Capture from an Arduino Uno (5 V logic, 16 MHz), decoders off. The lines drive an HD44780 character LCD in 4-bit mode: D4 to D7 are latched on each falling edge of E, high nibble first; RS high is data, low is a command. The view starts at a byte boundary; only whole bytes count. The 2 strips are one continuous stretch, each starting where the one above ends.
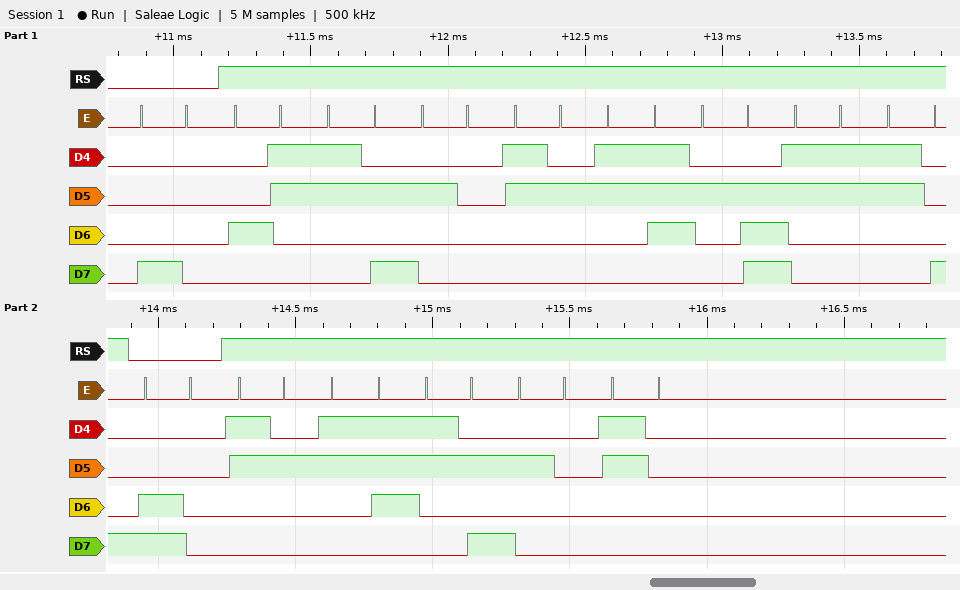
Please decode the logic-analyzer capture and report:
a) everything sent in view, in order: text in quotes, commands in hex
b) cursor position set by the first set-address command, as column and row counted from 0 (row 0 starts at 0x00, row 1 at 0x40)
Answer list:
0x80 "C: 27.38" 0xC0 "27: 0"
column 0, row 0
